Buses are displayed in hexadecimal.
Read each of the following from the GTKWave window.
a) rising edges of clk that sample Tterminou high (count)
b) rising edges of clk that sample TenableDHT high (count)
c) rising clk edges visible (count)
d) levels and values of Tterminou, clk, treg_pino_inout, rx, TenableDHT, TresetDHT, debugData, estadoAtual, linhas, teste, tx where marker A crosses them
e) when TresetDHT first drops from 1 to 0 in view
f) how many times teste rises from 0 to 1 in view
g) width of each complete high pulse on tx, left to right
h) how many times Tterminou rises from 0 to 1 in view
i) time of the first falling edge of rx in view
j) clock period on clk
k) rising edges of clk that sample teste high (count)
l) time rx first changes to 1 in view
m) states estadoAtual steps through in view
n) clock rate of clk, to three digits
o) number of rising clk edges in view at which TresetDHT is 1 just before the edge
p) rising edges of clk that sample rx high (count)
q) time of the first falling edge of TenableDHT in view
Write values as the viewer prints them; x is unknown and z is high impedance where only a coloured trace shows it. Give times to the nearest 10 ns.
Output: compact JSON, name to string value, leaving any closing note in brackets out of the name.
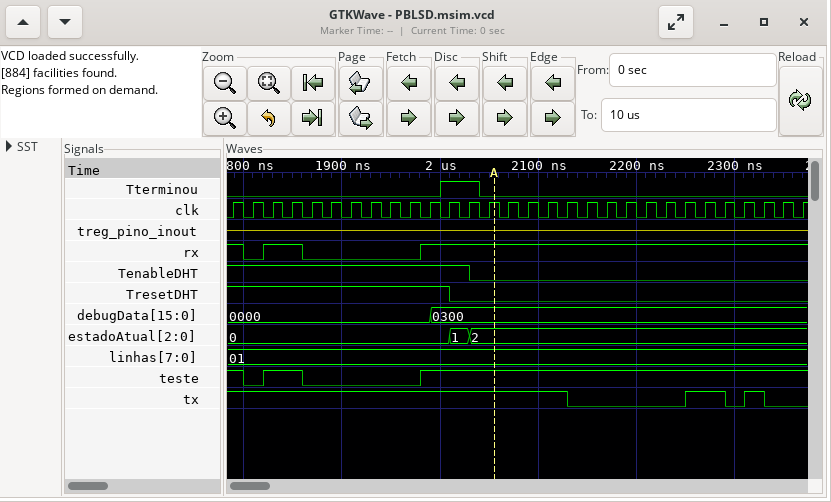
{"rising edges of clk that sample Tterminou high": "2", "rising edges of clk that sample TenableDHT high": "13", "rising clk edges visible": "30", "levels and values of Tterminou, clk, treg_pino_inout, rx, TenableDHT, TresetDHT, debugData, estadoAtual, linhas, teste, tx where marker A crosses them": "Tterminou=0, clk=1, treg_pino_inout=z, rx=1, TenableDHT=0, TresetDHT=0, debugData=0300, estadoAtual=2, linhas=01, teste=1, tx=1", "when TresetDHT first drops from 1 to 0 in view": "2010 ns", "how many times teste rises from 0 to 1 in view": "2", "width of each complete high pulse on tx, left to right": "40 ns, 20 ns", "how many times Tterminou rises from 0 to 1 in view": "1", "time of the first falling edge of rx in view": "1800 ns", "clock period on clk": "20 ns", "rising edges of clk that sample teste high": "23", "time rx first changes to 1 in view": "1820 ns", "states estadoAtual steps through in view": "0, 1, 2", "clock rate of clk, to three digits": "50.0 MHz", "number of rising clk edges in view at which TresetDHT is 1 just before the edge": "12", "rising edges of clk that sample rx high": "23", "time of the first falling edge of TenableDHT in view": "2030 ns"}
